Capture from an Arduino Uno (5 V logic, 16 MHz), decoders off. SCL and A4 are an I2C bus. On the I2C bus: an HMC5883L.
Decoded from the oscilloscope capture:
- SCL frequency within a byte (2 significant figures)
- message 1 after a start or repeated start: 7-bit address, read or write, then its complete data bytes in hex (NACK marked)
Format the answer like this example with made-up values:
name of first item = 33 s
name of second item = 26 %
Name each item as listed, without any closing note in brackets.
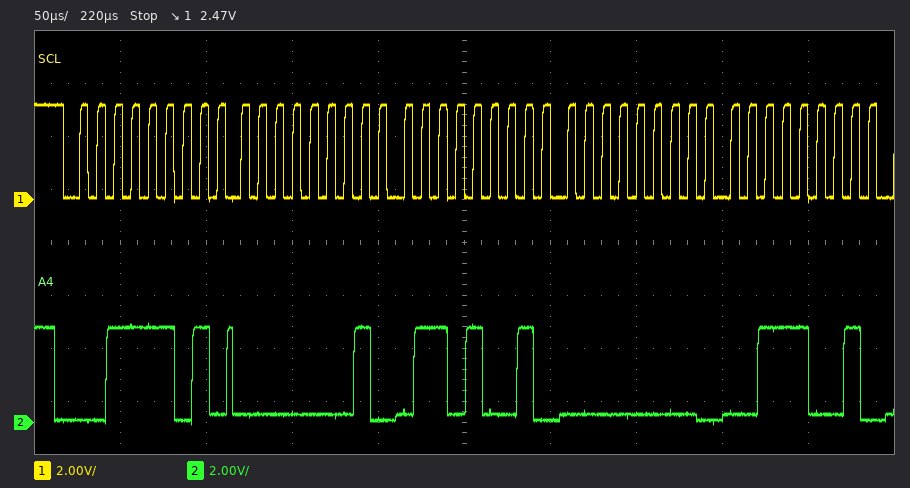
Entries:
SCL frequency within a byte = 100 kHz
message 1 after a start or repeated start: 7-bit address, read or write, then its complete data bytes in hex = 0x1E read: 01 69 00 39
